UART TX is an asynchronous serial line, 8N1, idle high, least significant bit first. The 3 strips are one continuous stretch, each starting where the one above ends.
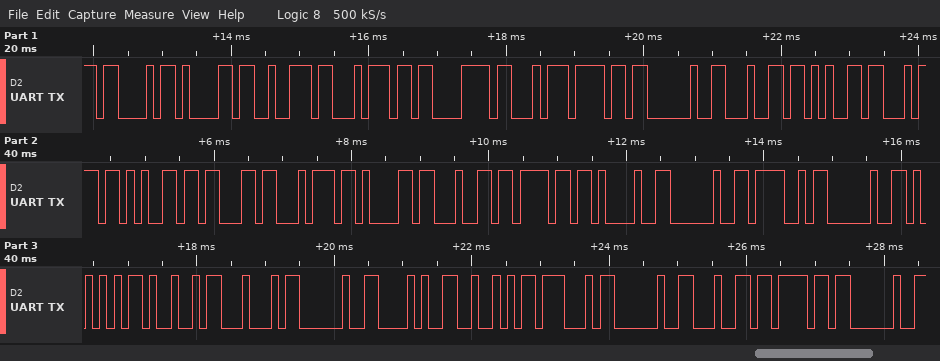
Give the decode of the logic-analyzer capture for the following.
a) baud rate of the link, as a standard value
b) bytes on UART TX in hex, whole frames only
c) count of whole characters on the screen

9600 baud
0x43 0x61 0x72 0x74 0xC3 0xA3 0x6F 0x20 0x64 0x65 0x74 0x65 0x63 0x74 0x61 0x64 0x6F 0x21 0x20 0x4F 0x20 0x55 0x49 0x44 0x20 0x28 0x52 0x47 0x20 0x64 0x6F 0x20
32
